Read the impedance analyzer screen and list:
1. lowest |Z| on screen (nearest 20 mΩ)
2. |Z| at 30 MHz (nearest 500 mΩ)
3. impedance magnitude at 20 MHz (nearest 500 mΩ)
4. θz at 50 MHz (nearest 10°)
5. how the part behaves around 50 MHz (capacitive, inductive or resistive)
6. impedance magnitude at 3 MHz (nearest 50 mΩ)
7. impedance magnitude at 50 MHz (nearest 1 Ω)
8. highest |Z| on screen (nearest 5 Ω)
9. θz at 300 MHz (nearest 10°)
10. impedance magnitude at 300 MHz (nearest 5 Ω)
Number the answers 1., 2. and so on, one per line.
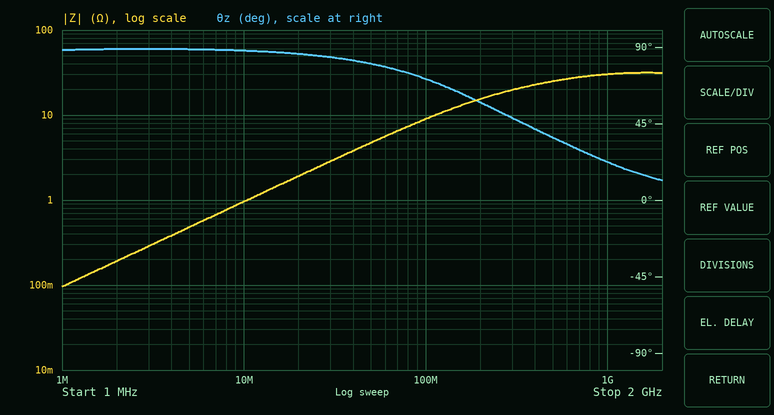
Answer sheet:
1. 100 mΩ
2. 3.0 Ω
3. 2.0 Ω
4. 80°
5. inductive
6. 300 mΩ
7. 5 Ω
8. 30 Ω
9. 50°
10. 20 Ω
